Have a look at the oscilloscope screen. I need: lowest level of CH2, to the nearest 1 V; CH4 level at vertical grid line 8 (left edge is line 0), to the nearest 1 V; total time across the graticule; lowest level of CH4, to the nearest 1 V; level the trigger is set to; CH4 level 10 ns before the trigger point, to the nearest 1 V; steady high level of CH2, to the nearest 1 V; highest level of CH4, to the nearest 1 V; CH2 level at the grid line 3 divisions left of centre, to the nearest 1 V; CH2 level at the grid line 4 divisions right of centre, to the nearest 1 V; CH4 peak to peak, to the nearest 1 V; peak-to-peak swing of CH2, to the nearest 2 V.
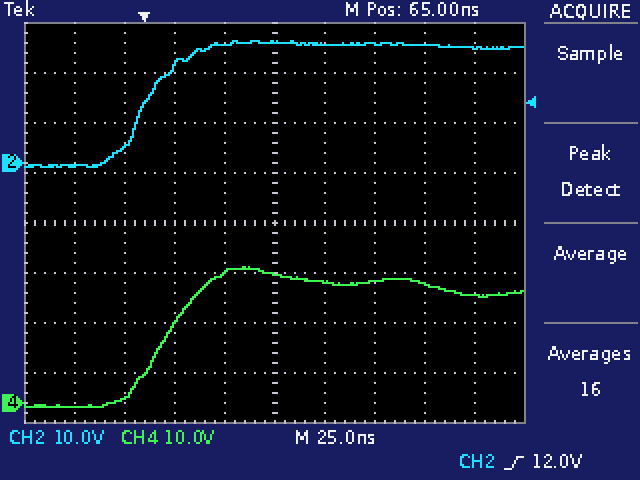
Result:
-1 V
24 V
250 ns
-1 V
12.0 V
1 V
24 V
27 V
3 V
23 V
28 V
26 V
